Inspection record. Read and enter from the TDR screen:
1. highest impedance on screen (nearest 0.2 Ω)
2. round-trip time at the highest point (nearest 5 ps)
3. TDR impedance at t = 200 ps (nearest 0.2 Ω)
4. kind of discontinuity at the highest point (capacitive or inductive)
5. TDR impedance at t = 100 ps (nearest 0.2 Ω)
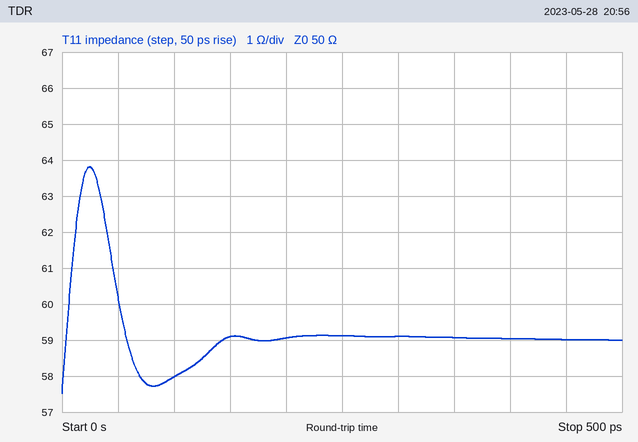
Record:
63.8 Ω
25 ps
59.0 Ω
inductive
58.0 Ω
